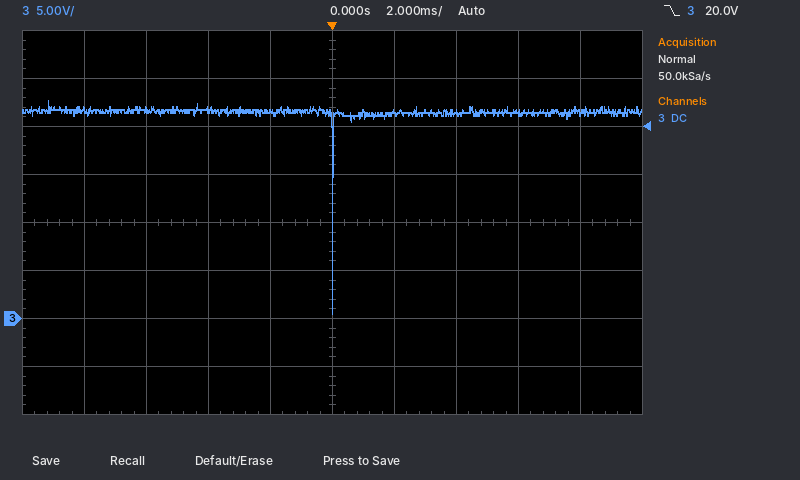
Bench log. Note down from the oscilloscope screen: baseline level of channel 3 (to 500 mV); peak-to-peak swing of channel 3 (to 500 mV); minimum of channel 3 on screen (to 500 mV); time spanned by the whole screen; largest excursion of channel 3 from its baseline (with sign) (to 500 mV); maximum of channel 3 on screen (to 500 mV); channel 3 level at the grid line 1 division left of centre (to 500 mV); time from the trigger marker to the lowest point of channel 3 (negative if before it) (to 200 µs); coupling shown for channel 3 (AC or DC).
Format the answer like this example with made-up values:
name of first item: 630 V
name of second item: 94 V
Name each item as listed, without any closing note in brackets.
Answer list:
baseline level of channel 3: 21.5 V
peak-to-peak swing of channel 3: 22.0 V
minimum of channel 3 on screen: 500 mV
time spanned by the whole screen: 20 ms
largest excursion of channel 3 from its baseline (with sign): -21.0 V
maximum of channel 3 on screen: 22.5 V
channel 3 level at the grid line 1 division left of centre: 21.5 V
time from the trigger marker to the lowest point of channel 3 (negative if before it): 0.0 ms
coupling shown for channel 3: DC
